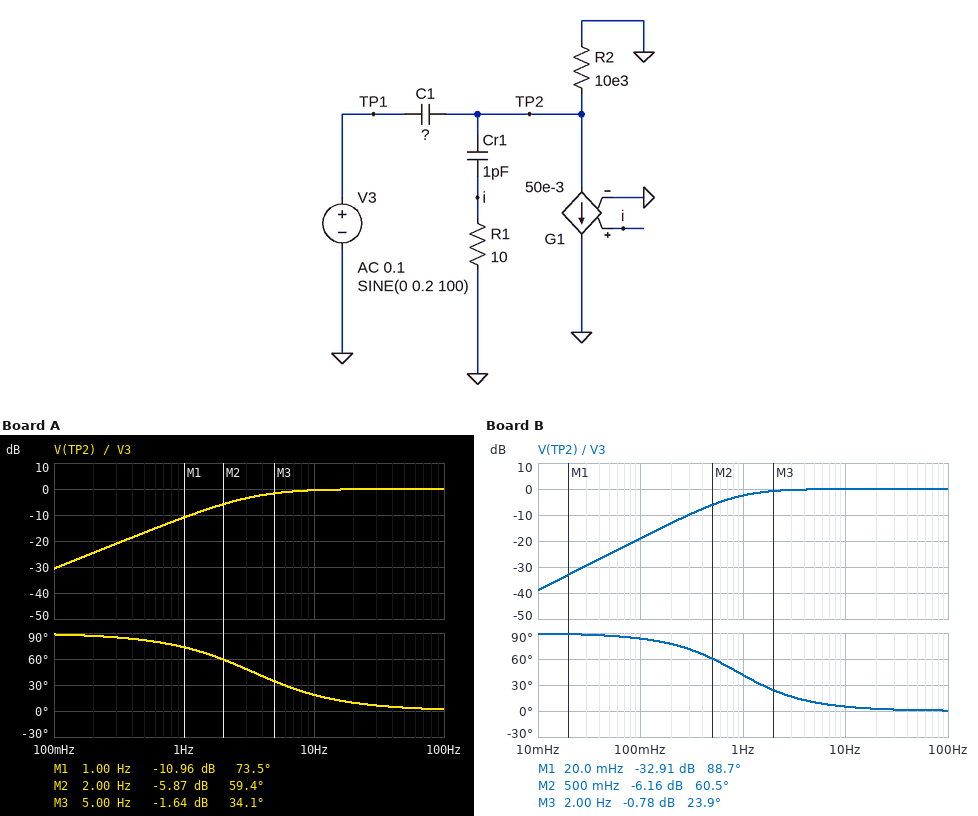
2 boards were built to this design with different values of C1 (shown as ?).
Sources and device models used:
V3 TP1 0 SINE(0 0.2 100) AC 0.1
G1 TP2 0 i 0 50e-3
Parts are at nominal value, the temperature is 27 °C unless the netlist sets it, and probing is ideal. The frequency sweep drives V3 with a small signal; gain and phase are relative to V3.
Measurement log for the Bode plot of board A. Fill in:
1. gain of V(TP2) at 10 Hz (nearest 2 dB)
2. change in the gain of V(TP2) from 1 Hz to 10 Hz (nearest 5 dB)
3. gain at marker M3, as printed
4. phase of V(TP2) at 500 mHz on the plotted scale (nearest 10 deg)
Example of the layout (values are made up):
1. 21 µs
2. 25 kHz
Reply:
1. 0 dB
2. 10 dB
3. -1.64 dB
4. 80 deg
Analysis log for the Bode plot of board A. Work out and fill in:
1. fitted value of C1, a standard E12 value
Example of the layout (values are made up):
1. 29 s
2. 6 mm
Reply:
1. 4.7 µF
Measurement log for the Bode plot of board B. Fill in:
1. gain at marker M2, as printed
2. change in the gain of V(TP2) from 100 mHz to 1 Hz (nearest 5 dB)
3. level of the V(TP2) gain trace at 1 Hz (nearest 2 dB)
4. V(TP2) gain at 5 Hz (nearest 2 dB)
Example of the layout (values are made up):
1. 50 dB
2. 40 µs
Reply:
1. -6.16 dB
2. 15 dB
3. -2 dB
4. 0 dB
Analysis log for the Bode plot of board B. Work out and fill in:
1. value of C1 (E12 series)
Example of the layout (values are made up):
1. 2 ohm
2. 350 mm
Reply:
1. 18 µF
